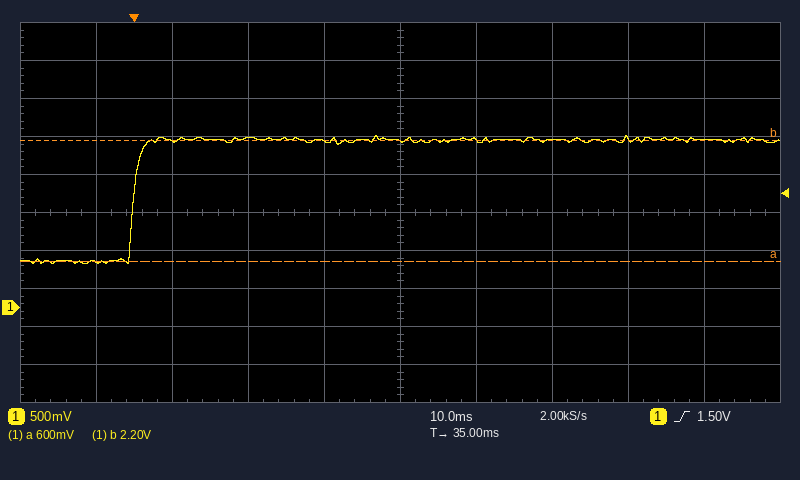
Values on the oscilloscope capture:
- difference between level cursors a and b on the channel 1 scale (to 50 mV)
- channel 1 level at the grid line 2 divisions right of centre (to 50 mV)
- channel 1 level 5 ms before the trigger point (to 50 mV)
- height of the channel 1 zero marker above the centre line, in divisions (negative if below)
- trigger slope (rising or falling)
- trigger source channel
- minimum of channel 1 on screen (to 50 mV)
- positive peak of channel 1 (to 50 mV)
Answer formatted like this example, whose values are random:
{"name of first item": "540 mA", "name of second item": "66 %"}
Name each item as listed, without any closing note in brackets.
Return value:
{"difference between level cursors a and b on the channel 1 scale": "1.60 V", "channel 1 level at the grid line 2 divisions right of centre": "2.20 V", "channel 1 level 5 ms before the trigger point": "600 mV", "height of the channel 1 zero marker above the centre line, in divisions": "-2.5 div", "trigger slope": "rising", "trigger source channel": "channel 1", "minimum of channel 1 on screen": "600 mV", "positive peak of channel 1": "2.25 V"}
